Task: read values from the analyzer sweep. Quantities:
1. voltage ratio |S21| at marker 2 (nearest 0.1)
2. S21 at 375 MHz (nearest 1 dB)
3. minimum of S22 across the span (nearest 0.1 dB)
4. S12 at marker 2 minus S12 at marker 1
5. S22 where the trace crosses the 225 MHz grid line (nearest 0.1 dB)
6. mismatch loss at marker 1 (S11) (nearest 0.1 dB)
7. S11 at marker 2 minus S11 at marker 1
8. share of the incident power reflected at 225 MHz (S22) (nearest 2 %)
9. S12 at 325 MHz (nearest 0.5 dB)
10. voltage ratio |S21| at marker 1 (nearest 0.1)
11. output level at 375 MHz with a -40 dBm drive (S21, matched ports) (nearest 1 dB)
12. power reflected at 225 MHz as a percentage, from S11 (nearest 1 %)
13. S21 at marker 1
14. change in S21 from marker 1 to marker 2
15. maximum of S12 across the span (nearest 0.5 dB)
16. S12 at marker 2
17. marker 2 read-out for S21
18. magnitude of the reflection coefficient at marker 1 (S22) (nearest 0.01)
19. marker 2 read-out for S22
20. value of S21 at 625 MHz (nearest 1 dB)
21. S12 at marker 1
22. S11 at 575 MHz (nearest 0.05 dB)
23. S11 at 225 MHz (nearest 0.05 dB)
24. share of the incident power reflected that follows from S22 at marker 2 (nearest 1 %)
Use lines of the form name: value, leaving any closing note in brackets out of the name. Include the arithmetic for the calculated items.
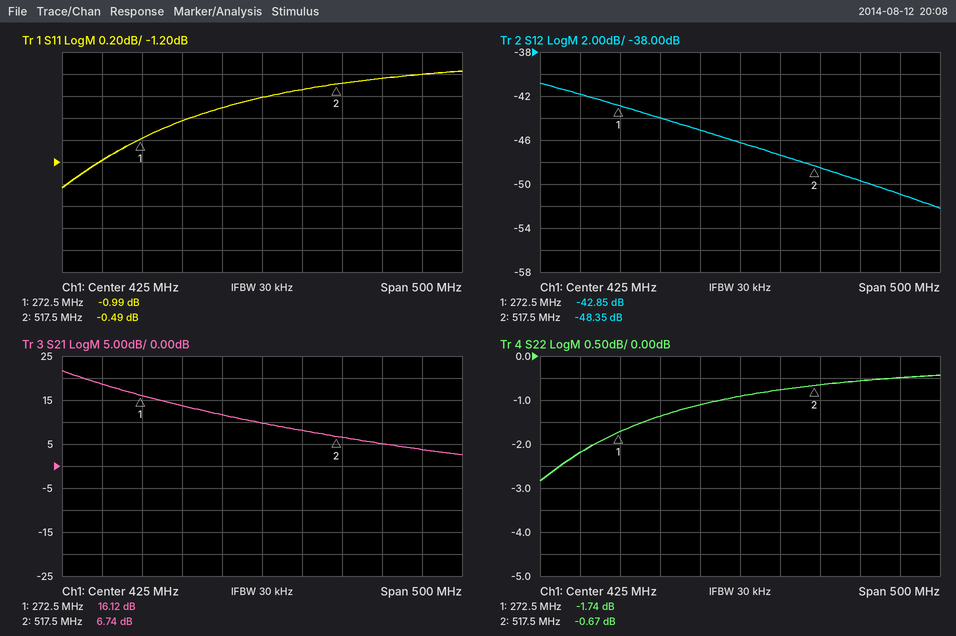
voltage ratio |S21| at marker 2: 10^(6.74/20) ≈ 2.2
S21 at 375 MHz: 12 dB
minimum of S22 across the span: -2.8 dB
S12 at marker 2 minus S12 at marker 1: -48.35 − (-42.85) = -5.50 dB
S22 where the trace crosses the 225 MHz grid line: -2.2 dB
mismatch loss at marker 1 (S11): −10 log10(1 − 10^(-0.99/10)) ≈ 6.9 dB
S11 at marker 2 minus S11 at marker 1: -0.49 − (-0.99) = 0.50 dB
share of the incident power reflected at 225 MHz (S22): 10^(-2.2/10) ≈ 60 %
S12 at 325 MHz: -44.0 dB
voltage ratio |S21| at marker 1: 10^(16.12/20) ≈ 6.4
output level at 375 MHz with a -40 dBm drive (S21, matched ports): -40 dBm + (12 dB) = -28 dBm
power reflected at 225 MHz as a percentage, from S11: 10^(-1.2/10) ≈ 76 %
S21 at marker 1: 16.12 dB
change in S21 from marker 1 to marker 2: 6.74 − (16.12) = -9.38 dB
maximum of S12 across the span: -41.0 dB
S12 at marker 2: -48.35 dB
marker 2 read-out for S21: 6.74 dB
magnitude of the reflection coefficient at marker 1 (S22): 10^(-1.74/20) ≈ 0.82
marker 2 read-out for S22: -0.67 dB
value of S21 at 625 MHz: 4 dB
S12 at marker 1: -42.85 dB
S11 at 575 MHz: -0.45 dB
S11 at 225 MHz: -1.20 dB
share of the incident power reflected that follows from S22 at marker 2: 10^(-0.67/10) ≈ 86 %
